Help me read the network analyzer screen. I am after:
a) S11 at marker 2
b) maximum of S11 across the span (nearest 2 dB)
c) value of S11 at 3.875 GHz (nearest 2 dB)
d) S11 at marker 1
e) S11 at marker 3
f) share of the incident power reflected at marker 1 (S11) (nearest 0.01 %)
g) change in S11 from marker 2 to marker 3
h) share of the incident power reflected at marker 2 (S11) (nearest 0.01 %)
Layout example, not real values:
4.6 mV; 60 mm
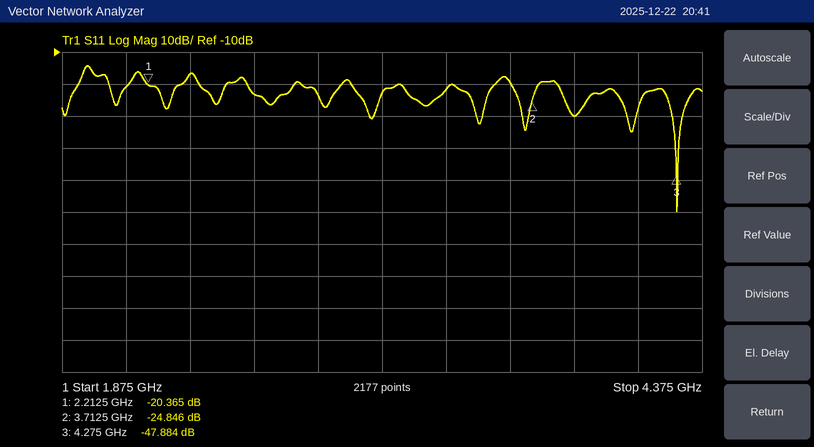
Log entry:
-24.846 dB; -14 dB; -30 dB; -20.365 dB; -47.884 dB; 0.92 %; -23.038 dB; 0.33 %
